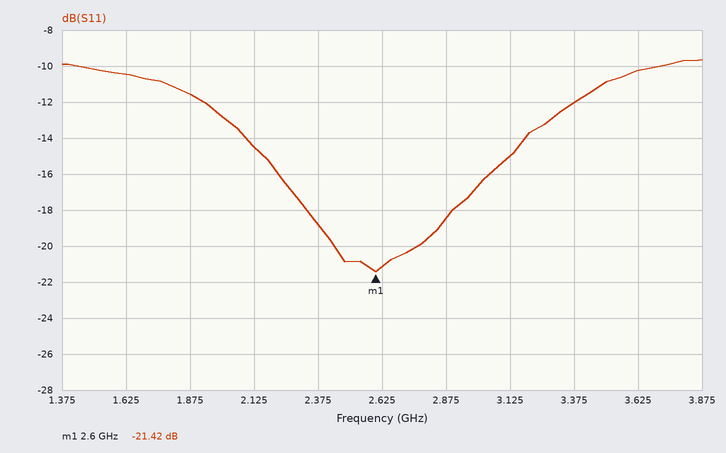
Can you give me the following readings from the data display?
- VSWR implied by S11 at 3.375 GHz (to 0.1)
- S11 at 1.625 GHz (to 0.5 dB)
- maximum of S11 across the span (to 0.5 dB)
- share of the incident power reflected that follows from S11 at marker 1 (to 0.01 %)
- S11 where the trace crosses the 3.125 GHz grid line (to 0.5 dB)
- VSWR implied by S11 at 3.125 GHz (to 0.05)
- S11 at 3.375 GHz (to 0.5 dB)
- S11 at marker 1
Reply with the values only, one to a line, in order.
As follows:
1.7
-10.5 dB
-9.5 dB
0.72 %
-15.0 dB
1.45
-12.0 dB
-21.42 dB
